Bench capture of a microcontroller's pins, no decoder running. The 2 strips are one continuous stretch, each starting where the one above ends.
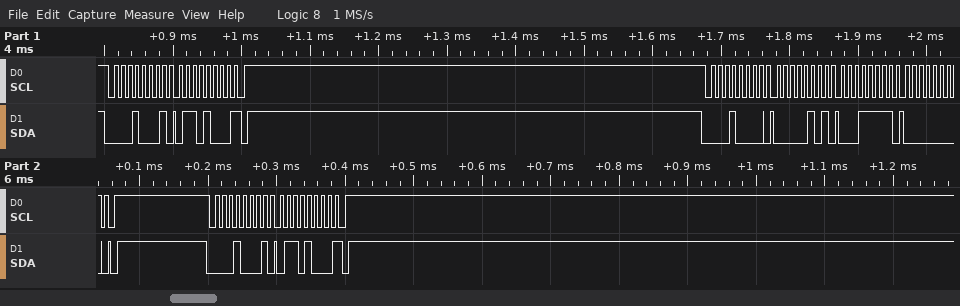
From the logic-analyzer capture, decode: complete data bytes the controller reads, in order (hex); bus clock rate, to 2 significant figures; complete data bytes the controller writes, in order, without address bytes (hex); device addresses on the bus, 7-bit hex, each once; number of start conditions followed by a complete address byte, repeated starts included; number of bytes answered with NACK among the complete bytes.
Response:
68 68
100 kHz
05 1F 00
0x08
3
2
